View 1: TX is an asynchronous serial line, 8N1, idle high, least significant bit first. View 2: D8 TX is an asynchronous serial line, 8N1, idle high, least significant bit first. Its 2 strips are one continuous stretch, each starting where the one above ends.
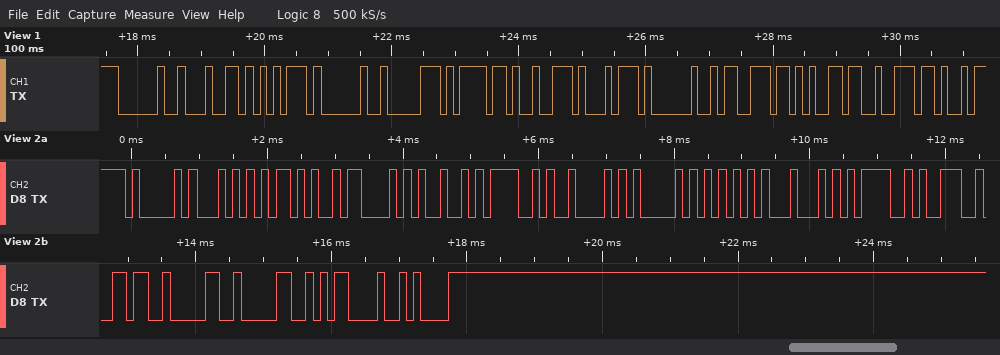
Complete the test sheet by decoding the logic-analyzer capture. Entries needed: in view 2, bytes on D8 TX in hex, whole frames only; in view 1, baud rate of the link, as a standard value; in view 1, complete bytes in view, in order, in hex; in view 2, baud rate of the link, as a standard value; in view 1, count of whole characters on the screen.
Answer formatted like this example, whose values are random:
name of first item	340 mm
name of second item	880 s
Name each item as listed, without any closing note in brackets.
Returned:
in view 2, bytes on D8 TX in hex, whole frames only	41 54 2B 43 49 4F 42 41 55 44 3D 39 36 30 30 0D 0A
in view 1, baud rate of the link, as a standard value	9600 baud
in view 1, complete bytes in view, in order, in hex	20 64 75 20 70 6F 72 74 20 73 65 72
in view 2, baud rate of the link, as a standard value	9600 baud
in view 1, count of whole characters on the screen	12
